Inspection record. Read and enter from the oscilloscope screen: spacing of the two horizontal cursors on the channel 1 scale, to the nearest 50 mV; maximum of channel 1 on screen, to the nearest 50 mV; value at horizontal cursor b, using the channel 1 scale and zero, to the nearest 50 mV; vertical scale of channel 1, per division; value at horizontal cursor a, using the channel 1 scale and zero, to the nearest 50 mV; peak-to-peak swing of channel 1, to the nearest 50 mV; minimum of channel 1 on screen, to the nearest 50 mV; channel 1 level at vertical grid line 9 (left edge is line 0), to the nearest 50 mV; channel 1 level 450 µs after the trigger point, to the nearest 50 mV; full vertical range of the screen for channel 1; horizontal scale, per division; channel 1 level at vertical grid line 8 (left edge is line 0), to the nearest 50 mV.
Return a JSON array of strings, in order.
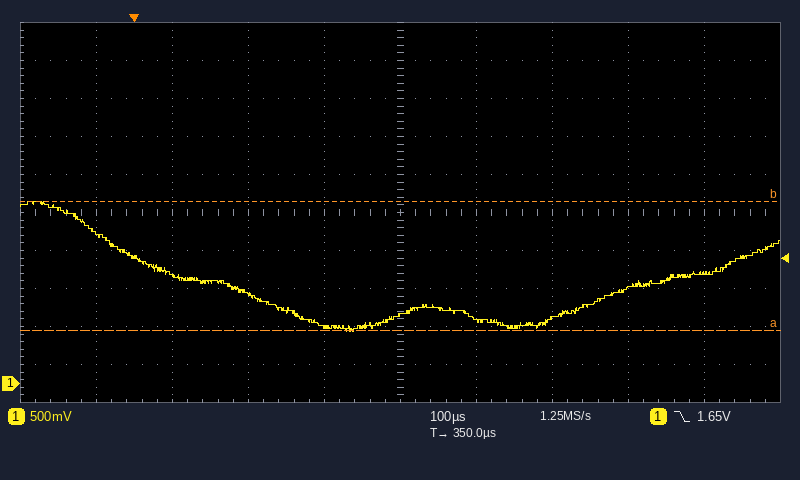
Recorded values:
["1.70 V", "2.40 V", "2.40 V", "500 mV", "700 mV", "1.70 V", "700 mV", "1.45 V", "850 mV", "5 V", "100 µs", "1.25 V"]
